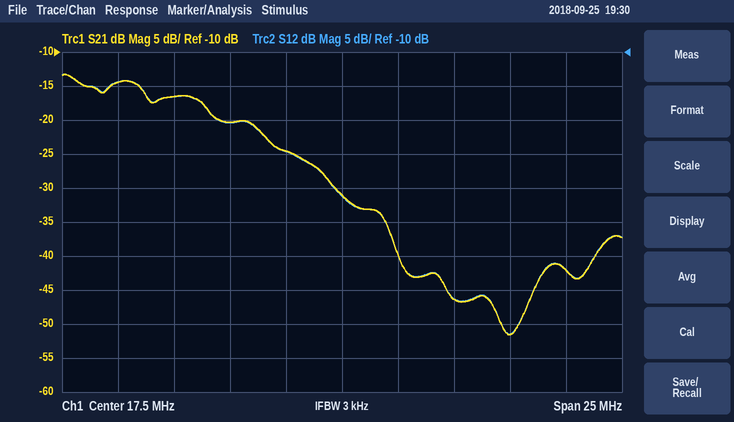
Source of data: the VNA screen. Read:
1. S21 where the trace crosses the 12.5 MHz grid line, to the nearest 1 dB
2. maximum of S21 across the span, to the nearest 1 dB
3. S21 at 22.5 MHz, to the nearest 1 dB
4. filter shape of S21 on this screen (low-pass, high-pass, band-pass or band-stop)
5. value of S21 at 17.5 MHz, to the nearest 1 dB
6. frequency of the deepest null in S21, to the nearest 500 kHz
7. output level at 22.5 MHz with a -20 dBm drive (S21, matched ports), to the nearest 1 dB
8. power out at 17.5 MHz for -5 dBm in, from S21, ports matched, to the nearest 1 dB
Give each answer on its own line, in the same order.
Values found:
-20 dB
-13 dB
-46 dB
low-pass
-31 dB
25.0 MHz
-66 dBm
-36 dBm
